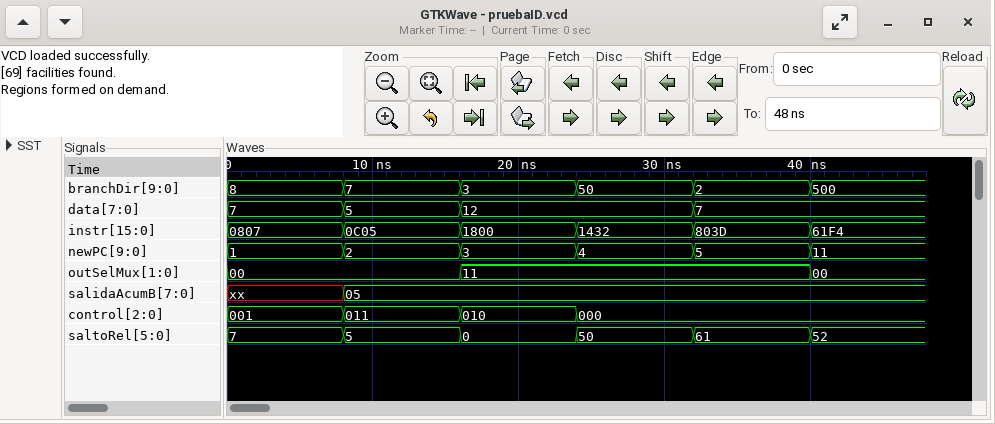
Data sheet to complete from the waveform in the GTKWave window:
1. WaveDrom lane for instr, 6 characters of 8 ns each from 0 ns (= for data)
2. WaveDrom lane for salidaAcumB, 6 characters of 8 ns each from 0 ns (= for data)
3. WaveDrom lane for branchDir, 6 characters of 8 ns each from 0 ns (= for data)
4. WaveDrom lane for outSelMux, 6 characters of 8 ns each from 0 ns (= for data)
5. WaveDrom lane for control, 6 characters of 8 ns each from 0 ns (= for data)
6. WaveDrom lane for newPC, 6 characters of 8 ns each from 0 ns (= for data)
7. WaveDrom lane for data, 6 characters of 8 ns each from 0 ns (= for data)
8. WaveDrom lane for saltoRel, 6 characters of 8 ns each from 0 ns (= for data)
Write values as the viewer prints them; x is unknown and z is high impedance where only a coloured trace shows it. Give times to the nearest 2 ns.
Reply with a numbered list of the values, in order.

1. {name: 'instr', wave: '======', data: '0807 0C05 1800 1432 803D 61F4'}
2. {name: 'salidaAcumB', wave: 'x=....', data: '05'}
3. {name: 'branchDir', wave: '======', data: '8 7 3 50 2 500'}
4. {name: 'outSelMux', wave: '=.=..=', data: '00 11 00'}
5. {name: 'control', wave: '====..', data: '001 011 010 000'}
6. {name: 'newPC', wave: '======', data: '1 2 3 4 5 11'}
7. {name: 'data', wave: '===.=.', data: '7 5 12 7'}
8. {name: 'saltoRel', wave: '======', data: '7 5 0 50 61 52'}
